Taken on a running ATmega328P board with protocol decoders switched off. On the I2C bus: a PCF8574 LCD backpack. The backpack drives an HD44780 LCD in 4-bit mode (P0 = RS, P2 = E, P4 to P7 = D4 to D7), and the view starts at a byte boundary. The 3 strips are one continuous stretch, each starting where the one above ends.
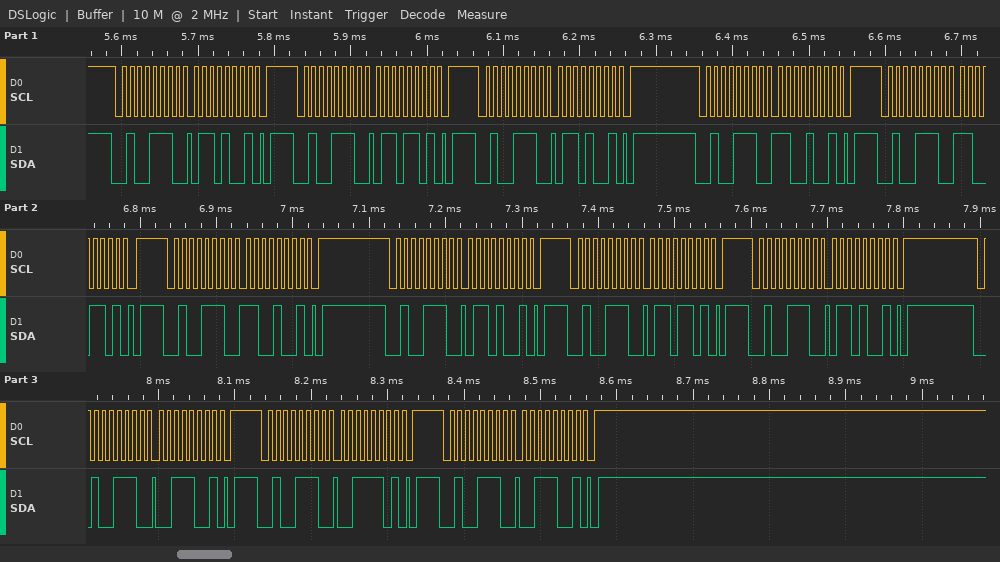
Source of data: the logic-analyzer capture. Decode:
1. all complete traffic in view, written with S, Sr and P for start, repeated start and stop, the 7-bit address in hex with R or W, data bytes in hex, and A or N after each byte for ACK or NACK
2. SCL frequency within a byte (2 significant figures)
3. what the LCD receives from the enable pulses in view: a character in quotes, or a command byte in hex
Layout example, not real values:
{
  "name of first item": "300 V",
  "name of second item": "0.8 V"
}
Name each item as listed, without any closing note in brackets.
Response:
{
  "all complete traffic in view, written with S, Sr and P for start, repeated start and stop, the 7-bit address in hex with R or W, data bytes in hex, and A or N after each byte for ACK or NACK": "S 27W A 69 A P S 27W A 6D A P S 27W A 69 A P S 27W A C9 A P S 27W A CD A P S 27W A C9 A P S 27W A 69 A P S 27W A 6D A P S 27W A 69 A P S 27W A 39 A P S 27W A 3D A P S 27W A 39 A P",
  "SCL frequency within a byte": "100 kHz",
  "what the LCD receives from the enable pulses in view: a character in quotes, or a command byte in hex": "'l' 'c'"
}
